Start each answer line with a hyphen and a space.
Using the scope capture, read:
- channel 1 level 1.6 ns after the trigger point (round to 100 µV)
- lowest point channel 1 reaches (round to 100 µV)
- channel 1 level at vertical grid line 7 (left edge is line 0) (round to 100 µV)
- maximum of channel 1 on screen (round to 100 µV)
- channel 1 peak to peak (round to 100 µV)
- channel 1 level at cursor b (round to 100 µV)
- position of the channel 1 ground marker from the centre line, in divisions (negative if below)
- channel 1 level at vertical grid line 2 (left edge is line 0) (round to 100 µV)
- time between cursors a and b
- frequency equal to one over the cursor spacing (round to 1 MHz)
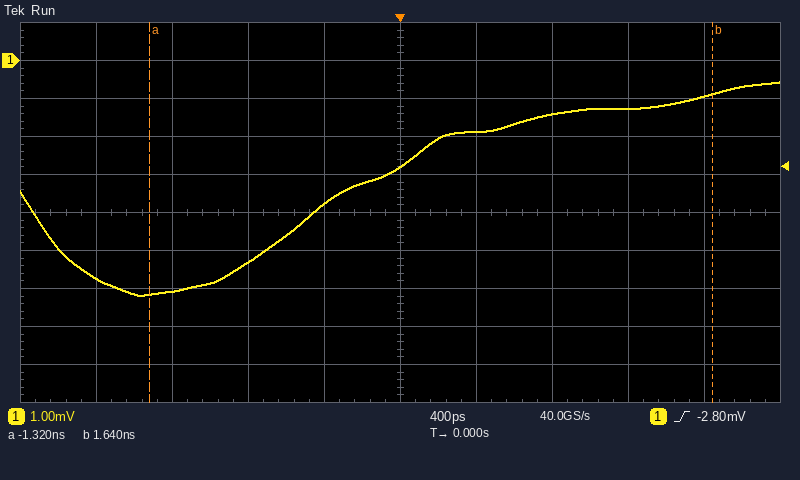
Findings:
- -900 µV
- -6.2 mV
- -1.4 mV
- -600 µV
- 5.6 mV
- -900 µV
- +4.0 div
- -6.1 mV
- 2.96 ns
- 338 MHz
